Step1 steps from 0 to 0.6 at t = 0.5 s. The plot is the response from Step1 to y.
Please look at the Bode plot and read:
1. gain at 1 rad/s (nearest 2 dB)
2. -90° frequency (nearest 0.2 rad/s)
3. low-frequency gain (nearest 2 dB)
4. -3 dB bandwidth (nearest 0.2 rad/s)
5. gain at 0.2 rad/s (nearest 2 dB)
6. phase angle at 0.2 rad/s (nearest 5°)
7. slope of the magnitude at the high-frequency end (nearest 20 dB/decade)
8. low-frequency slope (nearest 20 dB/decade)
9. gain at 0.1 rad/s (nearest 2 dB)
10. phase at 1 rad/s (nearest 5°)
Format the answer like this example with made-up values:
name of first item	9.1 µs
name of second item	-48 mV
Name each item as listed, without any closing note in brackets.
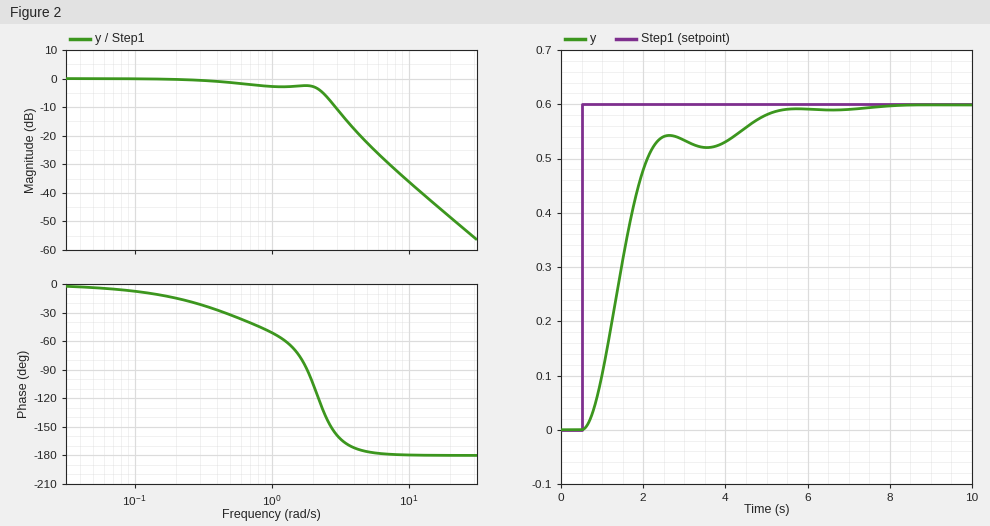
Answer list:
gain at 1 rad/s	-2 dB
-90° frequency	1.8 rad/s
low-frequency gain	0 dB
-3 dB bandwidth	2.0 rad/s
gain at 0.2 rad/s	0 dB
phase angle at 0.2 rad/s	-15°
slope of the magnitude at the high-frequency end	-40 dB/decade
low-frequency slope	0 dB/decade
gain at 0.1 rad/s	0 dB
phase at 1 rad/s	-50°
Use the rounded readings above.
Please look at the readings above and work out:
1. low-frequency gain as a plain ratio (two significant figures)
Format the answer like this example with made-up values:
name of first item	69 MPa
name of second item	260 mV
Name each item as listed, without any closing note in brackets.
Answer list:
low-frequency gain as a plain ratio	1.0
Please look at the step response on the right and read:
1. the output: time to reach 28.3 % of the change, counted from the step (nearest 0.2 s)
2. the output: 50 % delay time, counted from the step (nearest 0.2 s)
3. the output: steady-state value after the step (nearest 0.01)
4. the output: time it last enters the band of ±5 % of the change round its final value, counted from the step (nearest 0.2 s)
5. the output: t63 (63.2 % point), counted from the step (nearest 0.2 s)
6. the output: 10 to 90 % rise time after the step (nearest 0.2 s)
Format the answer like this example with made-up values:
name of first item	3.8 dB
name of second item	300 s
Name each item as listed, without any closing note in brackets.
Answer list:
the output: time to reach 28.3 % of the change, counted from the step	0.6 s
the output: 50 % delay time, counted from the step	1.0 s
the output: steady-state value after the step	0.60
the output: time it last enters the band of ±5 % of the change round its final value, counted from the step	4.2 s
the output: t63 (63.2 % point), counted from the step	1.2 s
the output: 10 to 90 % rise time after the step	1.6 s
